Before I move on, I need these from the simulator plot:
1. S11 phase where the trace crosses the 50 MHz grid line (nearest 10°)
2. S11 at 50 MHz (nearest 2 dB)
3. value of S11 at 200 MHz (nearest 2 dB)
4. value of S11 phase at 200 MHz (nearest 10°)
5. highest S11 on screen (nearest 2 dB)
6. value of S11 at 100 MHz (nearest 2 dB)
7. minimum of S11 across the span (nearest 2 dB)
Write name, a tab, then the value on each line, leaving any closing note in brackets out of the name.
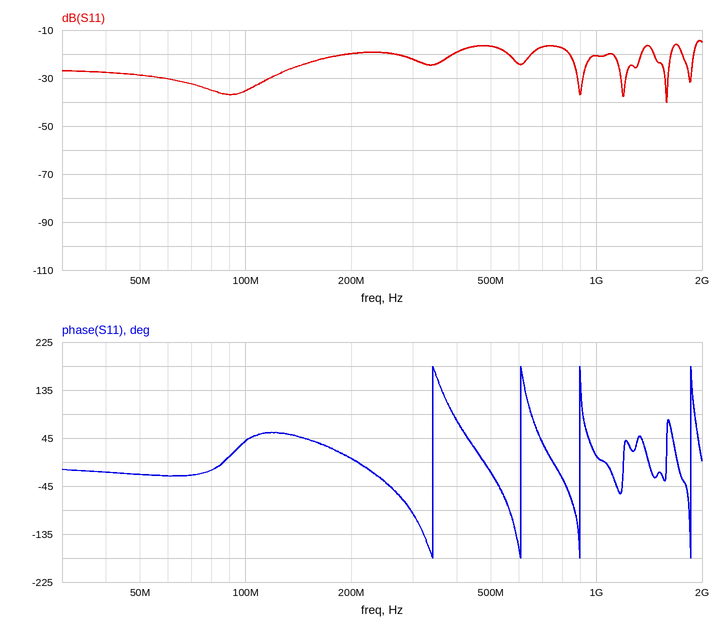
S11 phase where the trace crosses the 50 MHz grid line	-20°
S11 at 50 MHz	-28 dB
value of S11 at 200 MHz	-20 dB
value of S11 phase at 200 MHz	10°
highest S11 on screen	-14 dB
value of S11 at 100 MHz	-36 dB
minimum of S11 across the span	-40 dB
